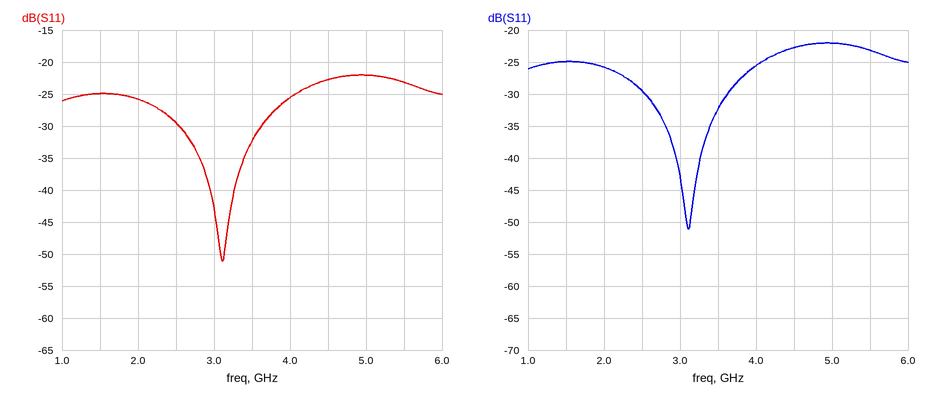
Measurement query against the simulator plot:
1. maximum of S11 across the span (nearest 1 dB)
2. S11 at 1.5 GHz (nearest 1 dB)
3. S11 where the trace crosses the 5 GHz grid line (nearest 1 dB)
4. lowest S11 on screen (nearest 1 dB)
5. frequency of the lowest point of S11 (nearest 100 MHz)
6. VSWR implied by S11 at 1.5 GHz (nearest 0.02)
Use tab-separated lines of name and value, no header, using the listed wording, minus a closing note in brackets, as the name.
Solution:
maximum of S11 across the span	-22 dB
S11 at 1.5 GHz	-25 dB
S11 where the trace crosses the 5 GHz grid line	-22 dB
lowest S11 on screen	-51 dB
frequency of the lowest point of S11	3.1 GHz
VSWR implied by S11 at 1.5 GHz	1.12
